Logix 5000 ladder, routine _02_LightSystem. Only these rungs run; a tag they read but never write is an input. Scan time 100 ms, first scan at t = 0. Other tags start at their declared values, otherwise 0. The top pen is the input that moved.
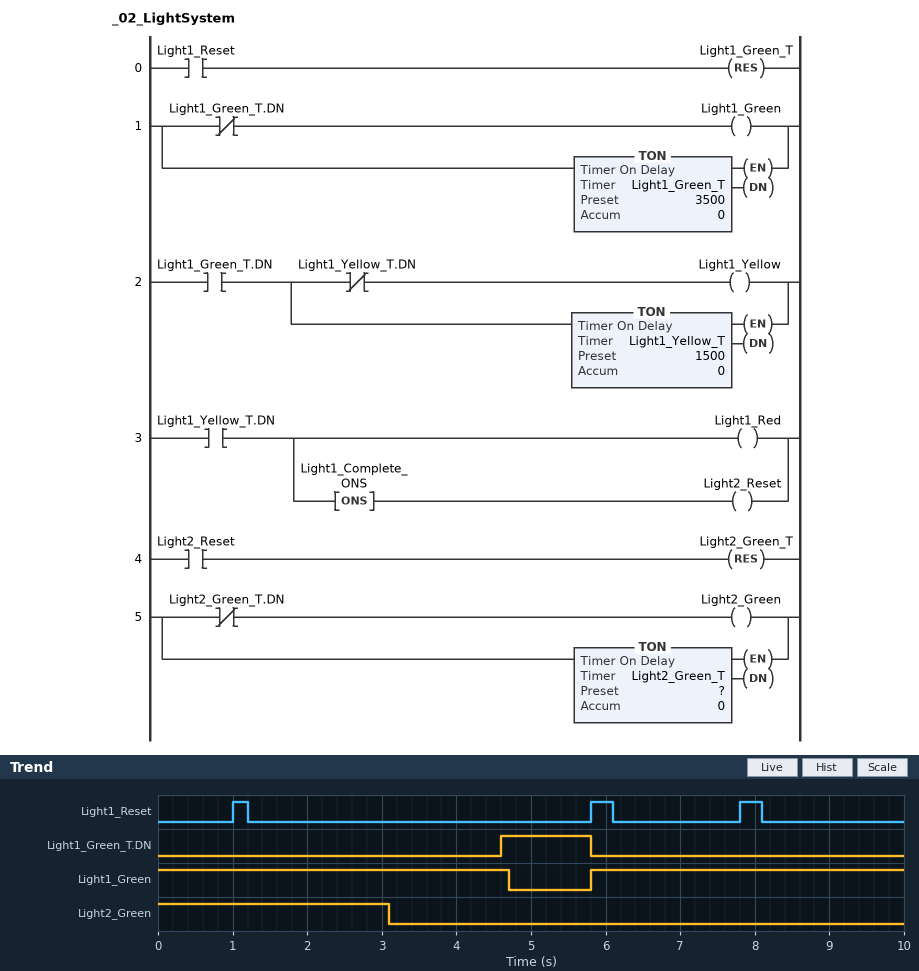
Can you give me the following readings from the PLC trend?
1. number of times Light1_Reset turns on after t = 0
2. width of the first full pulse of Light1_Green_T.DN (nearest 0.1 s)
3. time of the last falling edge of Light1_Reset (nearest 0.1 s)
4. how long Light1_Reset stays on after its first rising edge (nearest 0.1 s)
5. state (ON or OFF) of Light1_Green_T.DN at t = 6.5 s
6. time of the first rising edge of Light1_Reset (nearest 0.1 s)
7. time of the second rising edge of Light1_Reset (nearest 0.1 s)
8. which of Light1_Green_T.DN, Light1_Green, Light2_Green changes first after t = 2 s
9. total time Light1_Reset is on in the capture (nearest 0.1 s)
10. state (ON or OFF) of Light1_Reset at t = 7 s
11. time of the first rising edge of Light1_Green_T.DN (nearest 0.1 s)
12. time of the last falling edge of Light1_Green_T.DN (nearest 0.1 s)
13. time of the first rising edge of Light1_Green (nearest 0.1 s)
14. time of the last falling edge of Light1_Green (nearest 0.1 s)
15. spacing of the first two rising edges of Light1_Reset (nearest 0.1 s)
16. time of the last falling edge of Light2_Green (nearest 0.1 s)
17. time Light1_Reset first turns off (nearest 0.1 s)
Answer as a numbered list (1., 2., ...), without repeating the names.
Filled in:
1. 3
2. 1.2 s
3. 8.1 s
4. 0.2 s
5. OFF
6. 1.0 s
7. 5.8 s
8. Light2_Green
9. 0.8 s
10. OFF
11. 4.6 s
12. 5.8 s
13. 5.8 s
14. 4.7 s
15. 4.8 s
16. 3.1 s
17. 1.2 s
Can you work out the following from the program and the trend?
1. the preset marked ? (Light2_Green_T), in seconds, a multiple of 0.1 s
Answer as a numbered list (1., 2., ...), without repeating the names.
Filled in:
1. 3.0 s
